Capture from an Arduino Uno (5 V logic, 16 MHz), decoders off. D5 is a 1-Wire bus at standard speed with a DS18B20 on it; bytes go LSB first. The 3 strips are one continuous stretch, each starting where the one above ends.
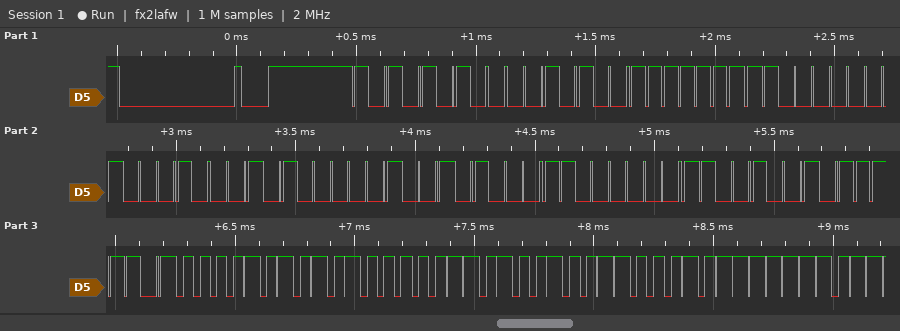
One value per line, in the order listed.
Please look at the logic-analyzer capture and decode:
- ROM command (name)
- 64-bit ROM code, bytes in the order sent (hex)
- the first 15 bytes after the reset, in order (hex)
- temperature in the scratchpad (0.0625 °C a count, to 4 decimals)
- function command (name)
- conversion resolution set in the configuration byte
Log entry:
Match ROM
28 FF 81 88 82 14 03 93
55 28 FF 81 88 82 14 03 93 BE 50 05 4B 46 7F
85.0000 °C
Read Scratchpad
12 bits
